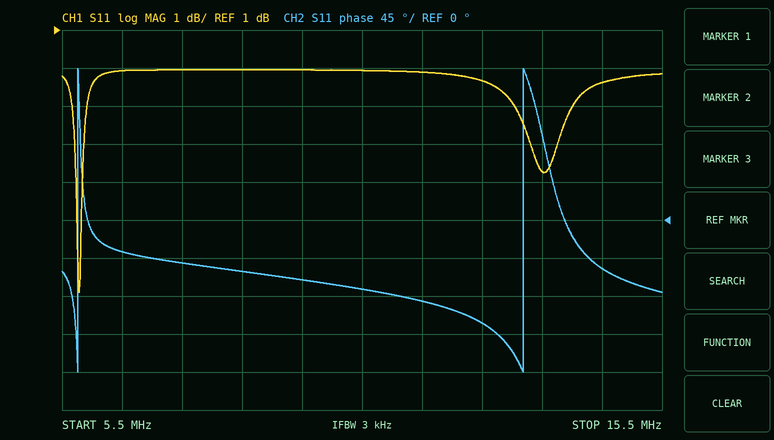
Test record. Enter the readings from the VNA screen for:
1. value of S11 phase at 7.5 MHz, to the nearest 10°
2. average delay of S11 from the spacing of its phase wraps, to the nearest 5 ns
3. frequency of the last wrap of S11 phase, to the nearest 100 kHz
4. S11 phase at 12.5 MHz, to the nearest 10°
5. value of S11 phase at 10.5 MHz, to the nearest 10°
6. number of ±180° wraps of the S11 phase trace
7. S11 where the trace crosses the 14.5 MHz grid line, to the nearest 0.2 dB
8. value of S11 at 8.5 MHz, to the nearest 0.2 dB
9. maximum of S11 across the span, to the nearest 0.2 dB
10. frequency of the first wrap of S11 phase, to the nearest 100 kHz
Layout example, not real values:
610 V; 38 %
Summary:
-50°; 135 ns; 13.2 MHz; -120°; -80°; 2; -0.4 dB; 0.0 dB; 0.0 dB; 5.8 MHz
